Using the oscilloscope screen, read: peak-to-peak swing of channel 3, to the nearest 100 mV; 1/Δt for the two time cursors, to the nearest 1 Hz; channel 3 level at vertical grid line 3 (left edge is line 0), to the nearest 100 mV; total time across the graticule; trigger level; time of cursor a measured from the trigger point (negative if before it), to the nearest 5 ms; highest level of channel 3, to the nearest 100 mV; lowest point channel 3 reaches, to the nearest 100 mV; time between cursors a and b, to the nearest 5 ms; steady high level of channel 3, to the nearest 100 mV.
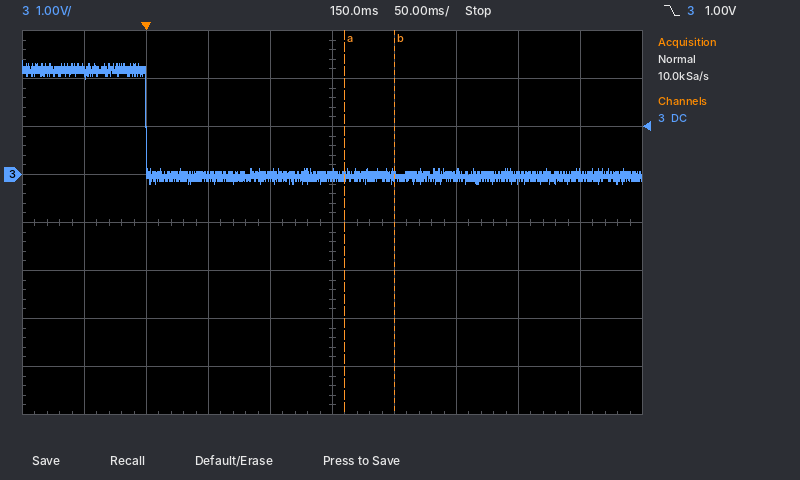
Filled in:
2.6 V
25 Hz
0.0 V
500 ms
1.00 V
+160 ms
2.4 V
-200 mV
40 ms
2.2 V
